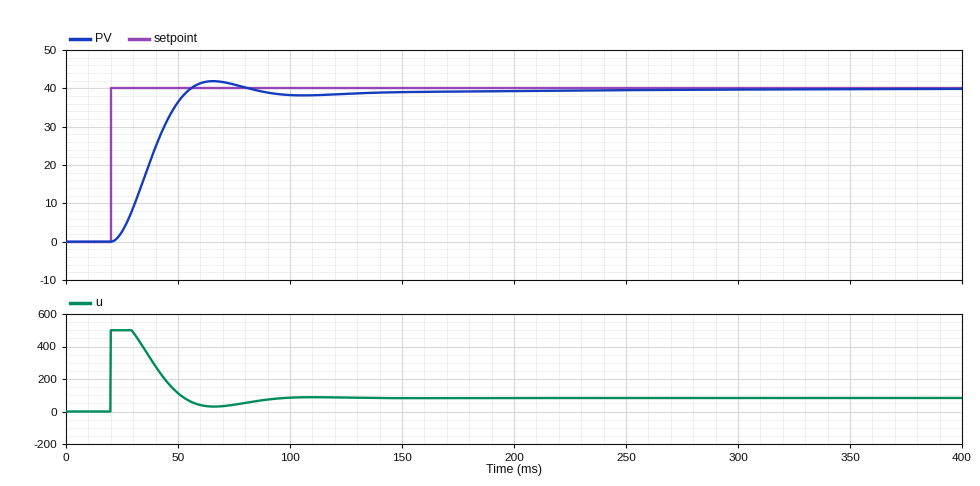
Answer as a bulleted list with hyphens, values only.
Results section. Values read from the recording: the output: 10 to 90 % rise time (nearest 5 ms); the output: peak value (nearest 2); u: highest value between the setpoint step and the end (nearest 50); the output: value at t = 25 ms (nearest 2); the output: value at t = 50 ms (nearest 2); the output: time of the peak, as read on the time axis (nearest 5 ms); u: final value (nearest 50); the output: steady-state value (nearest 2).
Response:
- 25 ms
- 42
- 500
- 2
- 36
- 65 ms
- 100
- 40
